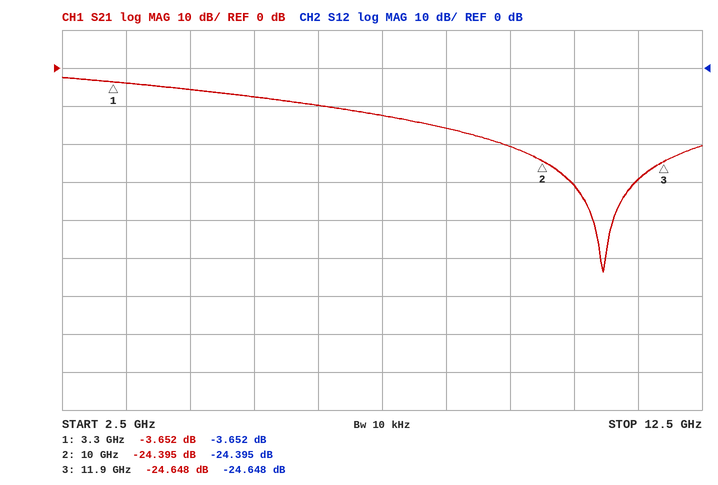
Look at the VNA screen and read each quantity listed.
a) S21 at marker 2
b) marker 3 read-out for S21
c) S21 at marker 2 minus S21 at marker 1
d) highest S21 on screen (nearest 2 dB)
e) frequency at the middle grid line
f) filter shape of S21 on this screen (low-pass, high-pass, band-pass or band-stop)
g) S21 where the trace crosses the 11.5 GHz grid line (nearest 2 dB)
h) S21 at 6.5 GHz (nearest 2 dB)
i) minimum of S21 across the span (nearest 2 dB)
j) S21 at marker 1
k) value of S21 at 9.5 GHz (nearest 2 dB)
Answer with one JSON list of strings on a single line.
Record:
["-24.395 dB", "-24.648 dB", "-20.743 dB", "-2 dB", "7.5 GHz", "low-pass", "-30 dB", "-10 dB", "-54 dB", "-3.652 dB", "-20 dB"]
